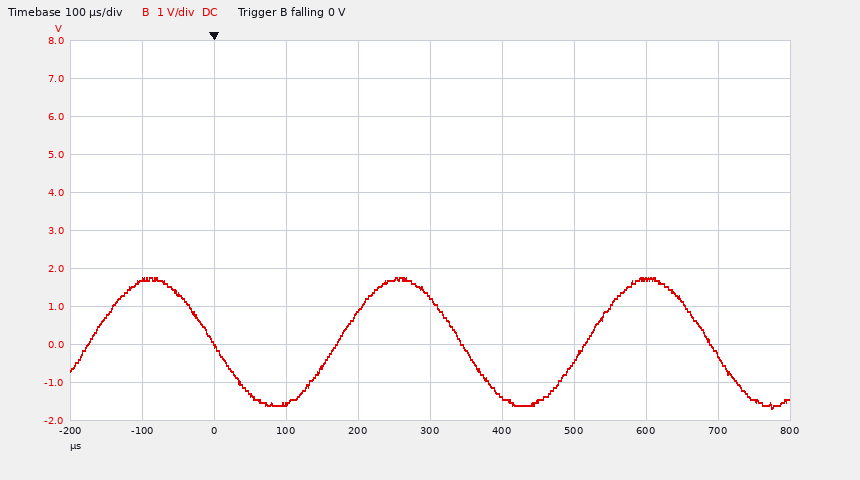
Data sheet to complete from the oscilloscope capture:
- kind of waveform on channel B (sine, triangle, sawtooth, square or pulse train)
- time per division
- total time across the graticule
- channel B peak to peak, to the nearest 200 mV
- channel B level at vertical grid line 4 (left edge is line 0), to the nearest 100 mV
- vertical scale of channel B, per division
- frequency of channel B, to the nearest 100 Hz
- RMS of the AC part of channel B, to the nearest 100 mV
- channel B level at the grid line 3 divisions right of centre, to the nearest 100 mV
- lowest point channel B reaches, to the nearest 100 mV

sine
100 µs
1 ms
3.4 V
900 mV
1 V
2.9 kHz
1.2 V
1.7 V
-1.7 V
